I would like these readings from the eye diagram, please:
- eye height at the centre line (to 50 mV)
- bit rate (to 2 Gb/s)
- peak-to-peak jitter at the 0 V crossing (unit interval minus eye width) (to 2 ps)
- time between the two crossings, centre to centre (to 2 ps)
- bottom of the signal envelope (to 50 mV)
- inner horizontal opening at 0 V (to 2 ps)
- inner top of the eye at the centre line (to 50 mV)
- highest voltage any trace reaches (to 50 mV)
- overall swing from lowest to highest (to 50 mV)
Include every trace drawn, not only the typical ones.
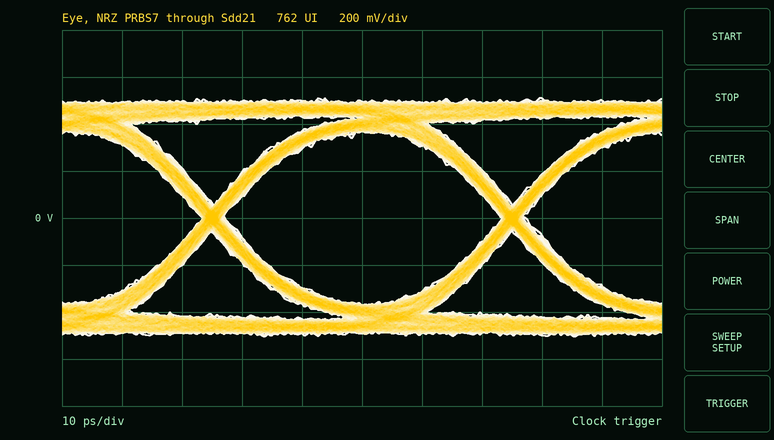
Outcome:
750 mV
20 Gb/s
4 ps
50 ps
-500 mV
46 ps
350 mV
500 mV
1.00 V
